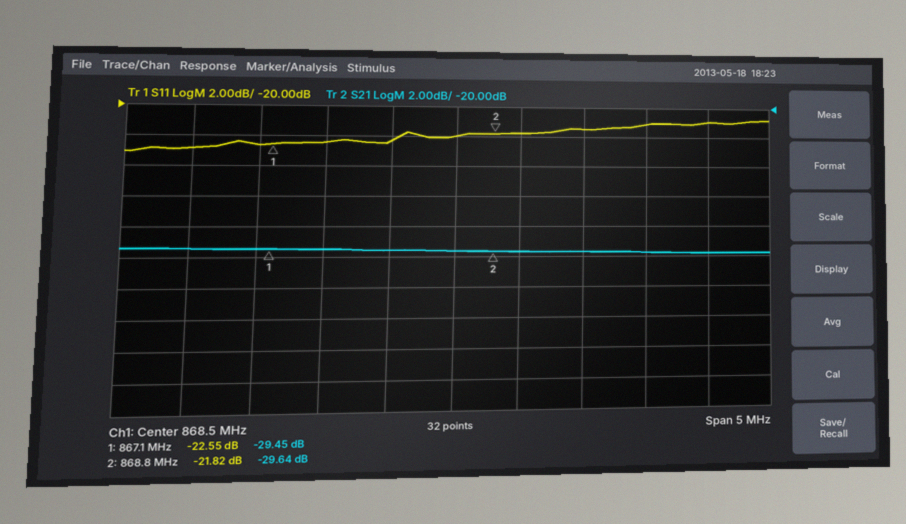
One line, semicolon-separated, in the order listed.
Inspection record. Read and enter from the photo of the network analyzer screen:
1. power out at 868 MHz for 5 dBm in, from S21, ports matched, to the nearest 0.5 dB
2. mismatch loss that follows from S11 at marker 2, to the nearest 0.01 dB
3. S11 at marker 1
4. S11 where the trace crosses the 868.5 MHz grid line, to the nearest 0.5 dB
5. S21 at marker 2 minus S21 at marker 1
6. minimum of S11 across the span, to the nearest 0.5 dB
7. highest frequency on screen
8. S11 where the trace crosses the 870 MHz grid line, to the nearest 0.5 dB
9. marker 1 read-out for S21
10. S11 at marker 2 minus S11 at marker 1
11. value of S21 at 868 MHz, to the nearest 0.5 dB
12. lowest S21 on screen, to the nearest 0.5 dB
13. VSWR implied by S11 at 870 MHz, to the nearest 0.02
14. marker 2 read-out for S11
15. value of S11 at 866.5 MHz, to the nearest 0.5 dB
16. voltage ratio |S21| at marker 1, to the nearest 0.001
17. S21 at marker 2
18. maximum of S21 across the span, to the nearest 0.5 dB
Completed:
-24.5 dBm; 0.03 dB; -22.55 dB; -22.0 dB; -0.19 dB; -23.0 dB; 871 MHz; -21.0 dB; -29.45 dB; 0.73 dB; -29.5 dB; -30.0 dB; 1.20; -21.82 dB; -23.0 dB; 0.034; -29.64 dB; -29.5 dB
